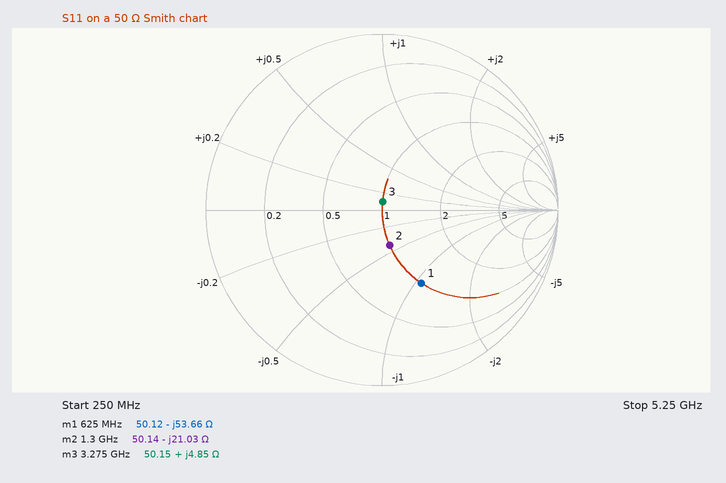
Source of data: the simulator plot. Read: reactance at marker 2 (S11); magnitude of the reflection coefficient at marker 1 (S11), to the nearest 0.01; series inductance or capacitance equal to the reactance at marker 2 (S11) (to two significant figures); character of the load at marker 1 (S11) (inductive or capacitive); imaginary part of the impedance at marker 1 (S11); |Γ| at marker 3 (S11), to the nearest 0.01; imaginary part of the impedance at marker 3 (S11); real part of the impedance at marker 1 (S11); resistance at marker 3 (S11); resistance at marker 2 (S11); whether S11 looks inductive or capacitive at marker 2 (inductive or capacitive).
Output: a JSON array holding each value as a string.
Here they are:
["-21.03 Ω", "0.47", "5.8 pF", "capacitive", "-53.66 Ω", "0.05", "+4.85 Ω", "50.12 Ω", "50.15 Ω", "50.14 Ω", "capacitive"]
